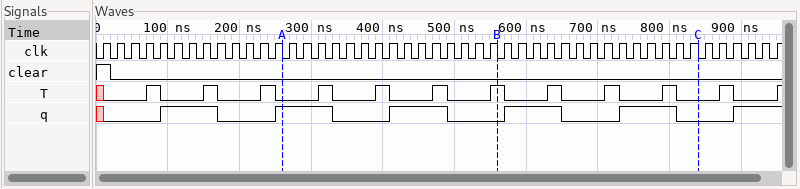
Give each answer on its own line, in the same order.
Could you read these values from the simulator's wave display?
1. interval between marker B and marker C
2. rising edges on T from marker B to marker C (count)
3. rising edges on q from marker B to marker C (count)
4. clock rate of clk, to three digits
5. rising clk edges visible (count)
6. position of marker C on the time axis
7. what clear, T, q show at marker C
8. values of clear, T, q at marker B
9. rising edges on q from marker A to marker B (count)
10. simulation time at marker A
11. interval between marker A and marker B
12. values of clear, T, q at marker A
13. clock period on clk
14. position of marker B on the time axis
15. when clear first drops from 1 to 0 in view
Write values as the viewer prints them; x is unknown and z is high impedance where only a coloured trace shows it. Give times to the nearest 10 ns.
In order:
280 ns
3
2
50.0 MHz
48
840 ns
clear=0, T=0, q=0
clear=0, T=1, q=0
1
260 ns
300 ns
clear=0, T=0, q=1
20 ns
560 ns
20 ns
